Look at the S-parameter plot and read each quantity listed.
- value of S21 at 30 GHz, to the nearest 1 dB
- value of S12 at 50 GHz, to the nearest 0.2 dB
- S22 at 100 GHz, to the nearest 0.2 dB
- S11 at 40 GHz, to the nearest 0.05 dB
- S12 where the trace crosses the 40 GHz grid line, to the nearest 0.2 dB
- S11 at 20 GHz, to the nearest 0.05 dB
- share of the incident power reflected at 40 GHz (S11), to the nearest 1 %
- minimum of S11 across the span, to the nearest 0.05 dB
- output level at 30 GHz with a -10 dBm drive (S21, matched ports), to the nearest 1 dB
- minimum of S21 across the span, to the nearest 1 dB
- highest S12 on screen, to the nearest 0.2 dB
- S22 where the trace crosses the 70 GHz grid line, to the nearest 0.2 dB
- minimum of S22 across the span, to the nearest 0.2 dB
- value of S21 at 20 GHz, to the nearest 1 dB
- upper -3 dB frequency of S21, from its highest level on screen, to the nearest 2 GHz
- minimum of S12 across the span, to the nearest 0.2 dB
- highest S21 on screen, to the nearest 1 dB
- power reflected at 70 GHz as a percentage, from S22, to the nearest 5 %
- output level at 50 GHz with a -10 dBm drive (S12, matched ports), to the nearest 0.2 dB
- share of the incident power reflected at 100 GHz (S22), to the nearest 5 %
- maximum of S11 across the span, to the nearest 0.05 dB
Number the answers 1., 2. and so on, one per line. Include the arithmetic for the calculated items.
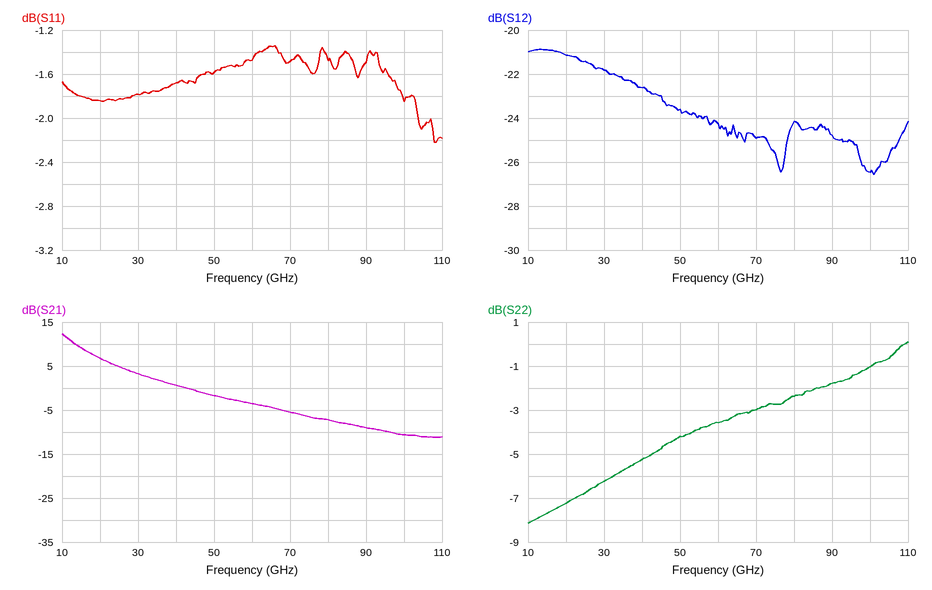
1. 3 dB
2. -23.6 dB
3. -1.0 dB
4. -1.70 dB
5. -22.6 dB
6. -1.85 dB
7. 10^(-1.7/10) ≈ 68 %
8. -2.20 dB
9. -10 dBm + (3 dB) = -7 dBm
10. -11 dB
11. -20.8 dB
12. -3.0 dB
13. -8.2 dB
14. 7 dB
15. 14 GHz
16. -26.6 dB
17. 12 dB
18. 10^(-3/10) ≈ 50 %
19. -10 dBm + (-23.6 dB) = -33.6 dBm
20. 10^(-1/10) ≈ 79.4 %, so 80 % to the nearest 5 %
21. -1.35 dB
